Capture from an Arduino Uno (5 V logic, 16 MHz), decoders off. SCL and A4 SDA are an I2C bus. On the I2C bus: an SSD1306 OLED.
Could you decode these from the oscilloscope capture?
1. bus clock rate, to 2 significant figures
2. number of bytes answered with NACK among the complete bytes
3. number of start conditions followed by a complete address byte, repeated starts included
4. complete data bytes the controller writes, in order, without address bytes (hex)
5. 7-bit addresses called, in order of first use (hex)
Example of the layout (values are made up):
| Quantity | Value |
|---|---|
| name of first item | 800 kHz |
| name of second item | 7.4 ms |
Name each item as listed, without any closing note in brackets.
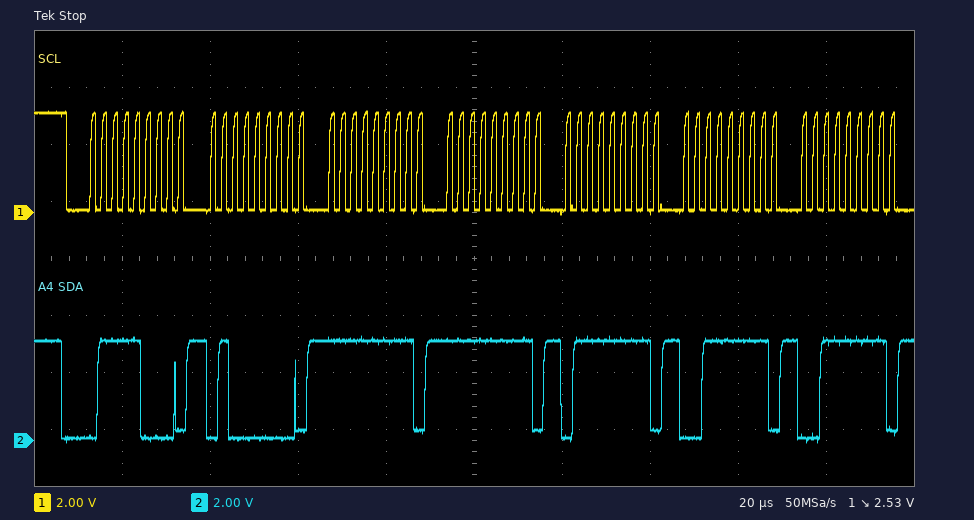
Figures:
| Quantity | Value |
|---|---|
| bus clock rate, to 2 significant figures | 400 kHz |
| number of bytes answered with NACK among the complete bytes | 0 |
| number of start conditions followed by a complete address byte, repeated starts included | 1 |
| complete data bytes the controller writes, in order, without address bytes | 40 FF FF 7F 3F 3F |
| 7-bit addresses called, in order of first use | 0x3C |
